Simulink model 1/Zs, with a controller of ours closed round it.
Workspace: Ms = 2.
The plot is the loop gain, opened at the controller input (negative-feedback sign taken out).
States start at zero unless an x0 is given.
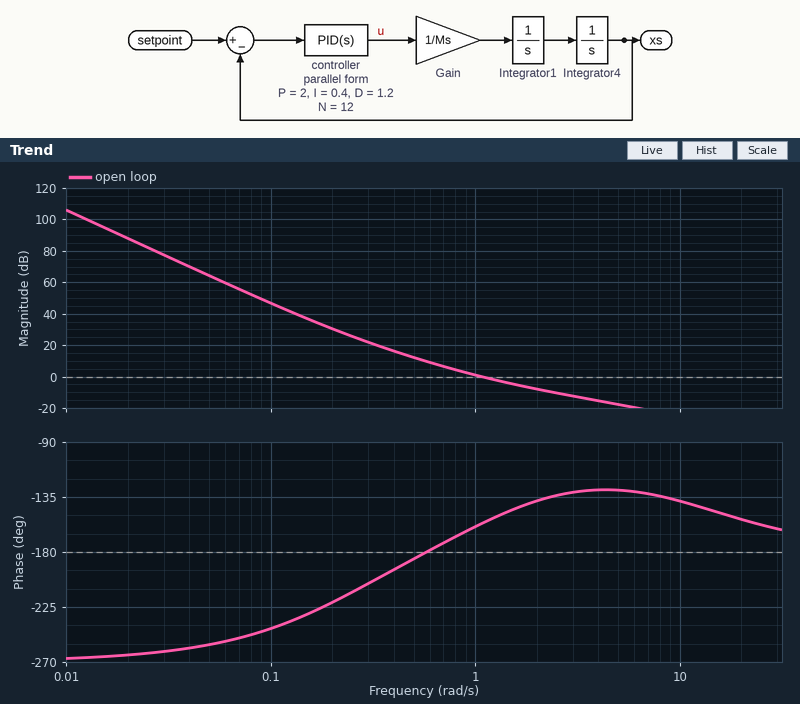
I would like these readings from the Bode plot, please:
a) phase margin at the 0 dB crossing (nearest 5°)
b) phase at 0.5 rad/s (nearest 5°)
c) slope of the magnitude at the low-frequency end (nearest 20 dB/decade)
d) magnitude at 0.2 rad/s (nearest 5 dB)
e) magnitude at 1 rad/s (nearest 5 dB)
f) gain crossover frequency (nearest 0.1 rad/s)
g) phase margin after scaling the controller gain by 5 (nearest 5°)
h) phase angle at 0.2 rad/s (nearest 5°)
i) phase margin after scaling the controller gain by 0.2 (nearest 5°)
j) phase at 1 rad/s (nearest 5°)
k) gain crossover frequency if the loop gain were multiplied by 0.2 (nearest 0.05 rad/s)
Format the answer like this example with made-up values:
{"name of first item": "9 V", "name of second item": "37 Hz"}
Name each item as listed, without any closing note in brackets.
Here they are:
{"phase margin at the 0 dB crossing": "25°", "phase at 0.5 rad/s": "-185°", "slope of the magnitude at the low-frequency end": "-60 dB/decade", "magnitude at 0.2 rad/s": "30 dB", "magnitude at 1 rad/s": "0 dB", "gain crossover frequency": "1.1 rad/s", "phase margin after scaling the controller gain by 5": "50°", "phase angle at 0.2 rad/s": "-220°", "phase margin after scaling the controller gain by 0.2": "-10°", "phase at 1 rad/s": "-160°", "gain crossover frequency if the loop gain were multiplied by 0.2": "0.45 rad/s"}
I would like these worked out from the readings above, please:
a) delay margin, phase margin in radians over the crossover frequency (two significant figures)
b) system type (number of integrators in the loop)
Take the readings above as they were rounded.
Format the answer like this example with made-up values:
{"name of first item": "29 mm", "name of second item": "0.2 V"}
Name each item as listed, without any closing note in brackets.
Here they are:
{"delay margin, phase margin in radians over the crossover frequency": "0.40 s", "system type": "3"}
